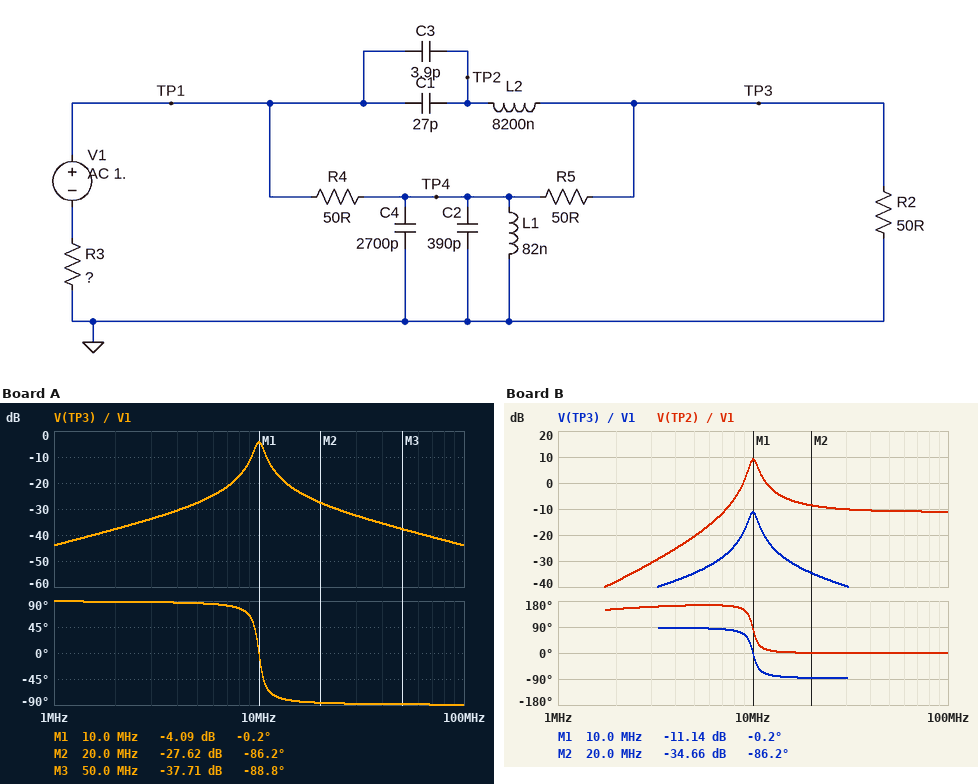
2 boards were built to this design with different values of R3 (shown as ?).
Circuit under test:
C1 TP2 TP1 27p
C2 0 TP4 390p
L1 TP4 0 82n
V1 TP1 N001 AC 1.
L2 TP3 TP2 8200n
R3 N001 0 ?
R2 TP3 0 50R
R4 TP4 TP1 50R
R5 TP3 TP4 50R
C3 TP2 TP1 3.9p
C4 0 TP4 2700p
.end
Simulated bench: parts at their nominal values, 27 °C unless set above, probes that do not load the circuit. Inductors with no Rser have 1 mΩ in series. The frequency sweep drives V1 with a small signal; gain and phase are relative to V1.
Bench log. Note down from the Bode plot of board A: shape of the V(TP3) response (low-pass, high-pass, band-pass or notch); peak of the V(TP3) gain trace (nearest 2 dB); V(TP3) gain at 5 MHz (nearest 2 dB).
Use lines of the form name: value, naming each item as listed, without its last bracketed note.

shape of the V(TP3) response: band-pass
peak of the V(TP3) gain trace: -4 dB
V(TP3) gain at 5 MHz: -28 dB
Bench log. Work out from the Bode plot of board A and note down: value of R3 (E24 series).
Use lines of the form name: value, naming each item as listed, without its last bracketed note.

value of R3: 30 Ω
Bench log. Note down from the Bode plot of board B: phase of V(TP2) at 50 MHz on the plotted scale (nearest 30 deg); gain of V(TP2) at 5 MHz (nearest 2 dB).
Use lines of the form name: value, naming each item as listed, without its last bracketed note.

phase of V(TP2) at 50 MHz on the plotted scale: 0 deg
gain of V(TP2) at 5 MHz: -20 dB
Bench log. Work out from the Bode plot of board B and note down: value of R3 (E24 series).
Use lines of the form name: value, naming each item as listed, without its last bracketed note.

value of R3: 130 Ω
